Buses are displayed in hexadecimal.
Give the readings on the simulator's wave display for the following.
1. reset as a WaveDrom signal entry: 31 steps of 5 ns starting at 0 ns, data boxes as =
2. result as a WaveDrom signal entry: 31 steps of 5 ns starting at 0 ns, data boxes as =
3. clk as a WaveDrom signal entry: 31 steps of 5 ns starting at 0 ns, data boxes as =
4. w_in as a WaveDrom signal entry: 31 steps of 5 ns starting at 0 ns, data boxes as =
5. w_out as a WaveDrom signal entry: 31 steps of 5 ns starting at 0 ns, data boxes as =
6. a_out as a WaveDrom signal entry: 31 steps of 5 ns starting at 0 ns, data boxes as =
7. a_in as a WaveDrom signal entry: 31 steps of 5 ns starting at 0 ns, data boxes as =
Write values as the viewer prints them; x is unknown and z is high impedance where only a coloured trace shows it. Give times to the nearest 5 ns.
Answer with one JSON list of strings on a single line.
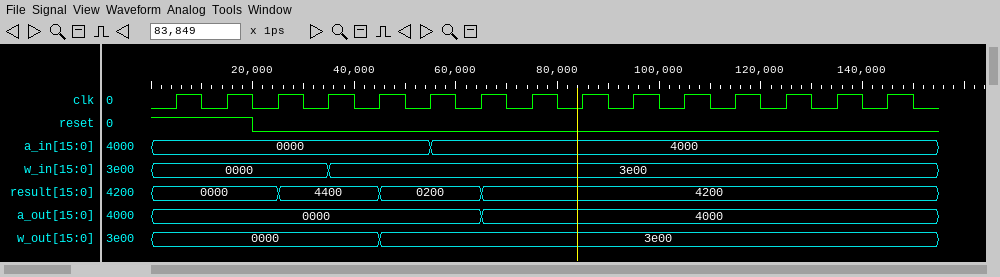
["{name: 'reset', wave: '1...0..........................'}", "{name: 'result', wave: '=....=...=...=.................', data: '0000 4400 0200 4200'}", "{name: 'clk', wave: '0101010101010101010101010101010'}", "{name: 'w_in', wave: '=......=.......................', data: '0000 3e00'}", "{name: 'w_out', wave: '=........=.....................', data: '0000 3e00'}", "{name: 'a_out', wave: '=............=.................', data: '0000 4000'}", "{name: 'a_in', wave: '=..........=...................', data: '0000 4000'}"]
